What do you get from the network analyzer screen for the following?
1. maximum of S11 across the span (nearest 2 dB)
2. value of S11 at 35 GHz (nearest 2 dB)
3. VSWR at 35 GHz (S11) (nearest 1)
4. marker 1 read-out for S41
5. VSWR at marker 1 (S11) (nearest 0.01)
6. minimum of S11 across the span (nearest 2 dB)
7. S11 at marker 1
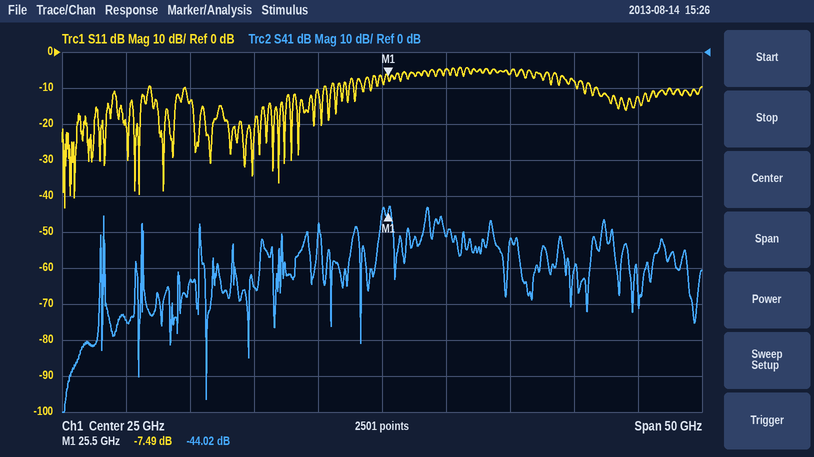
-4 dB
-6 dB
3
-44.02 dB
2.46
-44 dB
-7.49 dB
